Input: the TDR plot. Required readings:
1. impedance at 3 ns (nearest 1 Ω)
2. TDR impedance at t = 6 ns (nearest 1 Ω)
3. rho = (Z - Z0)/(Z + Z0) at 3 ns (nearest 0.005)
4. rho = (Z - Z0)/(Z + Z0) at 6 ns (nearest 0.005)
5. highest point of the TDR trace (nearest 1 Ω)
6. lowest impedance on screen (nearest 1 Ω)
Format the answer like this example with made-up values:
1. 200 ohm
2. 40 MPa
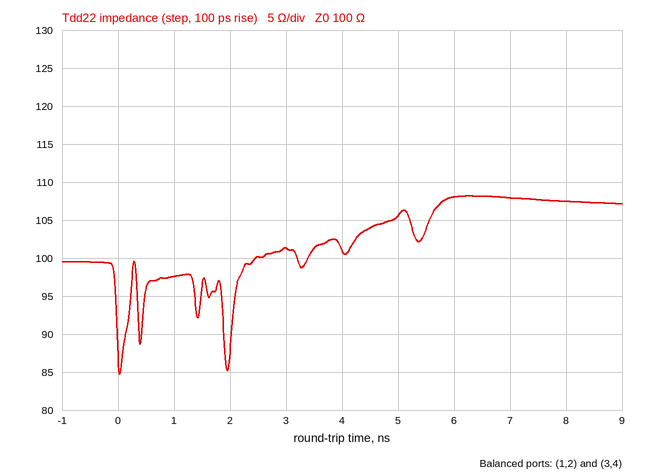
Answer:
1. 101 Ω
2. 108 Ω
3. +0.005
4. +0.040
5. 108 Ω
6. 85 Ω
